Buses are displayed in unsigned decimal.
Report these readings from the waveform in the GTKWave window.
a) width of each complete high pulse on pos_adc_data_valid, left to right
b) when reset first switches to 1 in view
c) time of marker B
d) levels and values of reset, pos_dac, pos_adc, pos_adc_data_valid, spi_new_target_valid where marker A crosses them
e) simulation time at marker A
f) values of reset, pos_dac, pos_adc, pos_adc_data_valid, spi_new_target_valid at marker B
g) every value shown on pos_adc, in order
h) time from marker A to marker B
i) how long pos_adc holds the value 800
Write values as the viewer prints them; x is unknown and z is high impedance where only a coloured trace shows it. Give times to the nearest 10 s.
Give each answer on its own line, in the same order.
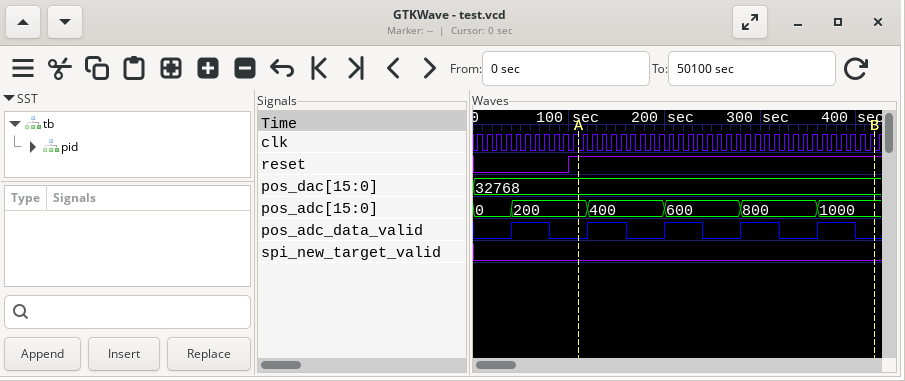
40 s, 40 s, 40 s, 40 s, 40 s
100 s
420 s
reset=1, pos_dac=32768, pos_adc=200, pos_adc_data_valid=0, spi_new_target_valid=0
110 s
reset=1, pos_dac=32768, pos_adc=1000, pos_adc_data_valid=0, spi_new_target_valid=0
0, 200, 400, 600, 800, 1000
310 s
80 s
